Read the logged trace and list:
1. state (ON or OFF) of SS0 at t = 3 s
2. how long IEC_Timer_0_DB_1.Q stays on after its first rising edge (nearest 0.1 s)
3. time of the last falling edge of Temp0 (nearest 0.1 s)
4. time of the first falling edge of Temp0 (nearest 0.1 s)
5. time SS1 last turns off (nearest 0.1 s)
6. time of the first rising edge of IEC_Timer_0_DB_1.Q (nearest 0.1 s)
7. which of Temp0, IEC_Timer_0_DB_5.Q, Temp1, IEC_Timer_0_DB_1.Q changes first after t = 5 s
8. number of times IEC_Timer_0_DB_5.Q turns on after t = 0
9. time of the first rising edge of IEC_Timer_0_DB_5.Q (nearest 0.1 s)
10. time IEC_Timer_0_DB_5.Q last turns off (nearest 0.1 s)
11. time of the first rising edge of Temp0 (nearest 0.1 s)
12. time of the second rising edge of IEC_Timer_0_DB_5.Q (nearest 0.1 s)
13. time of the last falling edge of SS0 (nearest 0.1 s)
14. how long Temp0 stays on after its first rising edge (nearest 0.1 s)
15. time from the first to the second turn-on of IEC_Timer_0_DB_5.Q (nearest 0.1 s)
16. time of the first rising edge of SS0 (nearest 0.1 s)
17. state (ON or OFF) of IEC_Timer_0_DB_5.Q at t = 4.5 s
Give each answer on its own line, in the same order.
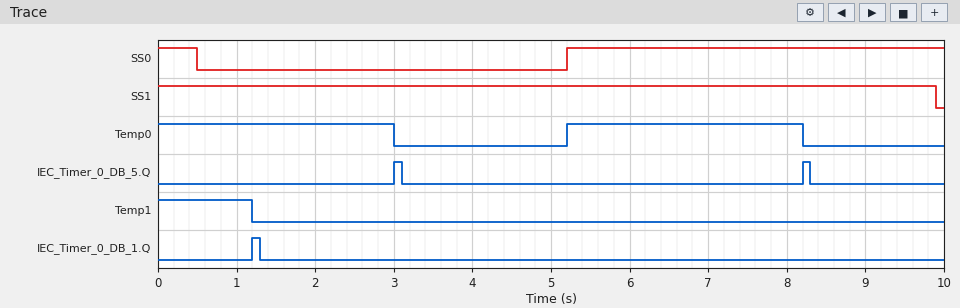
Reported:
OFF
0.1 s
8.2 s
3.0 s
9.9 s
1.2 s
Temp0
2
3.0 s
8.3 s
5.2 s
8.2 s
0.5 s
3.0 s
5.2 s
5.2 s
OFF
